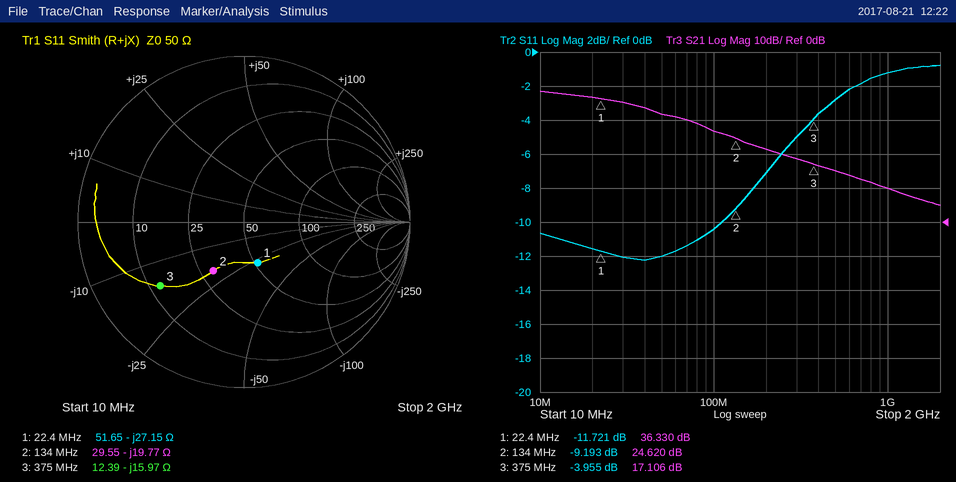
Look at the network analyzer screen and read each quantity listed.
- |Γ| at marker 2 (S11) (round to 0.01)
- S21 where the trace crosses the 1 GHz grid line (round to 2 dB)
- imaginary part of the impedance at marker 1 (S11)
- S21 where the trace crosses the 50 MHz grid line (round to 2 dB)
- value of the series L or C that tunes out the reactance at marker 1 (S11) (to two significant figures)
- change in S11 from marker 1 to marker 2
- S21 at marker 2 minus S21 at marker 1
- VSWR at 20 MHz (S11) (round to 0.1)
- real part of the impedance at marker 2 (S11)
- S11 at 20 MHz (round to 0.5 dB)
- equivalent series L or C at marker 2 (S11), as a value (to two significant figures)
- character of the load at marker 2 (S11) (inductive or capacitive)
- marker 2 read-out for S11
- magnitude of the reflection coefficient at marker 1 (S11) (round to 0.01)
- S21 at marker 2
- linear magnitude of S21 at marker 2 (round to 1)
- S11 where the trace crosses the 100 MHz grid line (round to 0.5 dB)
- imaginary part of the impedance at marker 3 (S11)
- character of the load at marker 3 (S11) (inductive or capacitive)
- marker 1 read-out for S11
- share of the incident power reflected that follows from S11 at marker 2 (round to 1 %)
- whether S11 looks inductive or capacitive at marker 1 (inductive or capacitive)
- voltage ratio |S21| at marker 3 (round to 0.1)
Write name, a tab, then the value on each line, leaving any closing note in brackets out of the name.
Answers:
|Γ| at marker 2 (S11)	0.35
S21 where the trace crosses the 1 GHz grid line	10 dB
imaginary part of the impedance at marker 1	-27.15 Ω
S21 where the trace crosses the 50 MHz grid line	32 dB
value of the series L or C that tunes out the reactance at marker 1 (S11)	190 nH
change in S11 from marker 1 to marker 2	2.528 dB
S21 at marker 2 minus S21 at marker 1	-11.710 dB
VSWR at 20 MHz (S11)	1.7
real part of the impedance at marker 2	29.55 Ω
S11 at 20 MHz	-11.5 dB
equivalent series L or C at marker 2 (S11), as a value	60 pF
character of the load at marker 2 (S11)	capacitive
marker 2 read-out for S11	-9.193 dB
magnitude of the reflection coefficient at marker 1 (S11)	0.26
S21 at marker 2	24.620 dB
linear magnitude of S21 at marker 2	17
S11 where the trace crosses the 100 MHz grid line	-10.5 dB
imaginary part of the impedance at marker 3	-15.97 Ω
character of the load at marker 3 (S11)	capacitive
marker 1 read-out for S11	-11.721 dB
share of the incident power reflected that follows from S11 at marker 2	12 %
whether S11 looks inductive or capacitive at marker 1	capacitive
voltage ratio |S21| at marker 3	7.2
